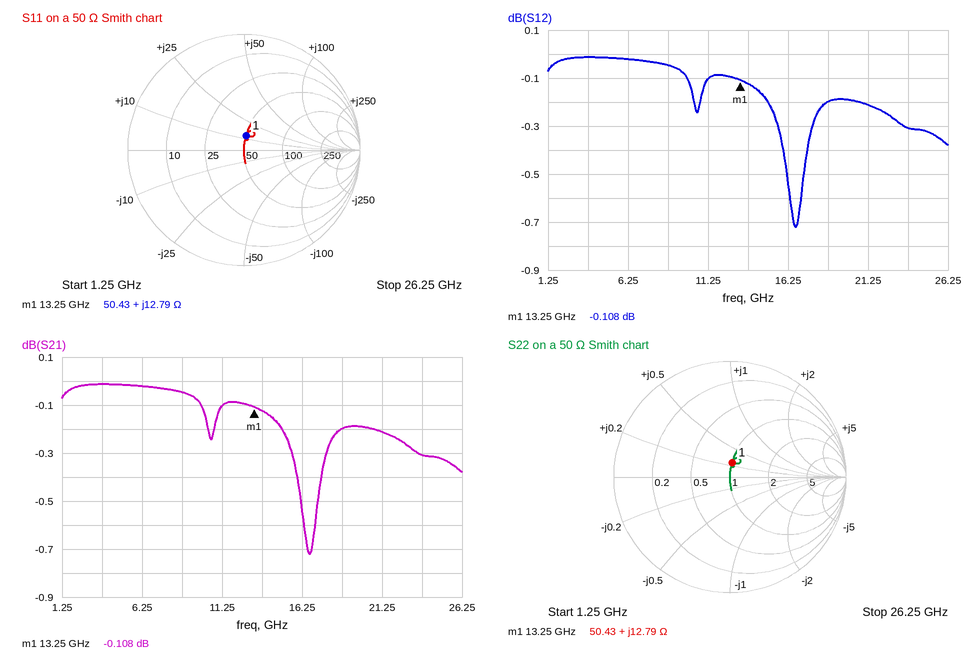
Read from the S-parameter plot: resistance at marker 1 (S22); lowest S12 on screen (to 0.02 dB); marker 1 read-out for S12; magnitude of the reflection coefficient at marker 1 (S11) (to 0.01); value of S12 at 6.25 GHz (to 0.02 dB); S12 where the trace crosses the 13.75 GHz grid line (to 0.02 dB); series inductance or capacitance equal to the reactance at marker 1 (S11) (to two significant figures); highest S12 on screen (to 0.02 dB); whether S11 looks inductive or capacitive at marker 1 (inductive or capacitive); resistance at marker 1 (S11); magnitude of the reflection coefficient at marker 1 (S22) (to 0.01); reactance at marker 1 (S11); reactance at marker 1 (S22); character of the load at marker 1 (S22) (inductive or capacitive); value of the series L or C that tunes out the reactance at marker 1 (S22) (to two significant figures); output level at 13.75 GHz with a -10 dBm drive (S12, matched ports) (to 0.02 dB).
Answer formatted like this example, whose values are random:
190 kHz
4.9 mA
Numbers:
50.43 Ω
-0.72 dB
-0.108 dB
0.13
-0.02 dB
-0.12 dB
150 pH
-0.02 dB
inductive
50.43 Ω
0.13
+12.79 Ω
+12.79 Ω
inductive
940 fF
-10.12 dBm
